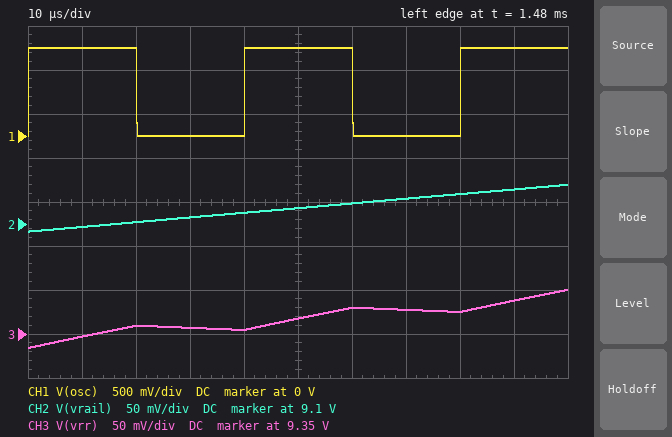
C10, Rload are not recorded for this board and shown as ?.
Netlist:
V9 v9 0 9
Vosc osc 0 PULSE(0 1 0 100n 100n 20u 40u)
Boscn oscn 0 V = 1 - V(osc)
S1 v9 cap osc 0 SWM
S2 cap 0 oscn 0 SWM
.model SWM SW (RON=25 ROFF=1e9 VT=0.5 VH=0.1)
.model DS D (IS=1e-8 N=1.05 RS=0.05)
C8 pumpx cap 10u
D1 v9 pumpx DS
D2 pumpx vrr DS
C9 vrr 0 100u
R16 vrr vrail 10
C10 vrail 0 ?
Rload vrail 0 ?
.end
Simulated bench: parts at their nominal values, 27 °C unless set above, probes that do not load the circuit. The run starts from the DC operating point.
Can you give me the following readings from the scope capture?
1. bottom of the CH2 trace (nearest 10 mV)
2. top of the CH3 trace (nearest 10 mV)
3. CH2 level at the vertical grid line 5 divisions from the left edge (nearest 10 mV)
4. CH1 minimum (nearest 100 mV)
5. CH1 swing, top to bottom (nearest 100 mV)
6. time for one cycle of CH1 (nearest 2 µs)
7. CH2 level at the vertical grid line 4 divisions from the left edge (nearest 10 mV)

9.09 V
9.40 V
9.12 V
0 V
1.0 V
40 µs
9.11 V
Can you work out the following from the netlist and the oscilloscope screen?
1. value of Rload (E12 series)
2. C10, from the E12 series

2.2 kΩ
39 µF
